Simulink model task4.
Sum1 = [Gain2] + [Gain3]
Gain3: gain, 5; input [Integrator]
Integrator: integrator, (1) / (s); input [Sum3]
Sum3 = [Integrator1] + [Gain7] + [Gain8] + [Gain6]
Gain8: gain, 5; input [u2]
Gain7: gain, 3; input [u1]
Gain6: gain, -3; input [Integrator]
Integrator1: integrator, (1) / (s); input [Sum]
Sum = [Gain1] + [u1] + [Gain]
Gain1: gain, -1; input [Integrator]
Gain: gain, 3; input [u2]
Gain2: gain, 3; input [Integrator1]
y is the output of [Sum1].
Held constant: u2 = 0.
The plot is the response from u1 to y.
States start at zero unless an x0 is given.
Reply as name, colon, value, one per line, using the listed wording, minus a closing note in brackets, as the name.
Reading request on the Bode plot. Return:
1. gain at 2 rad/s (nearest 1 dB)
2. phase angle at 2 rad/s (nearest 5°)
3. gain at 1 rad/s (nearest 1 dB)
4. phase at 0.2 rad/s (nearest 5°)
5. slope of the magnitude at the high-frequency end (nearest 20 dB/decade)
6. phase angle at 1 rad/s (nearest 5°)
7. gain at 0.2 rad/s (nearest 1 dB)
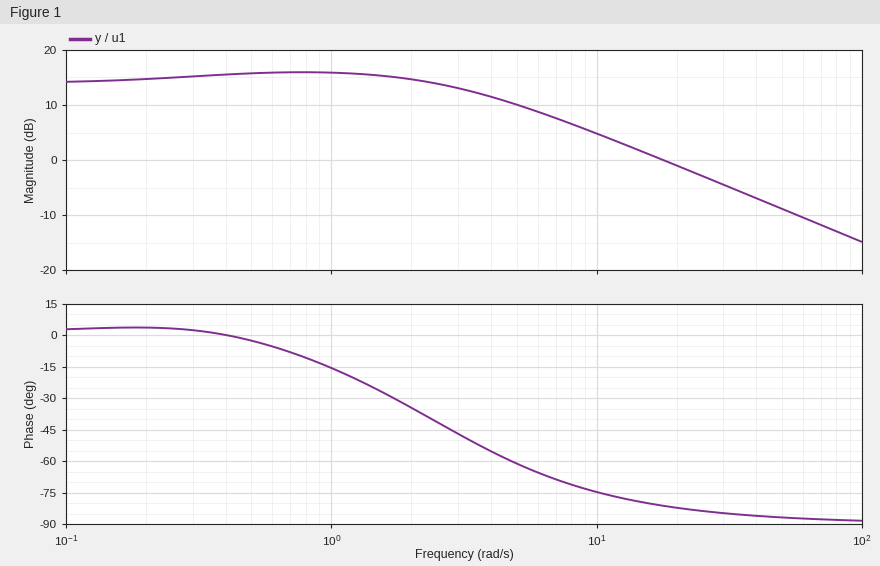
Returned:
gain at 2 rad/s: 15 dB
phase angle at 2 rad/s: -35°
gain at 1 rad/s: 16 dB
phase at 0.2 rad/s: 5°
slope of the magnitude at the high-frequency end: -20 dB/decade
phase angle at 1 rad/s: -15°
gain at 0.2 rad/s: 15 dB
